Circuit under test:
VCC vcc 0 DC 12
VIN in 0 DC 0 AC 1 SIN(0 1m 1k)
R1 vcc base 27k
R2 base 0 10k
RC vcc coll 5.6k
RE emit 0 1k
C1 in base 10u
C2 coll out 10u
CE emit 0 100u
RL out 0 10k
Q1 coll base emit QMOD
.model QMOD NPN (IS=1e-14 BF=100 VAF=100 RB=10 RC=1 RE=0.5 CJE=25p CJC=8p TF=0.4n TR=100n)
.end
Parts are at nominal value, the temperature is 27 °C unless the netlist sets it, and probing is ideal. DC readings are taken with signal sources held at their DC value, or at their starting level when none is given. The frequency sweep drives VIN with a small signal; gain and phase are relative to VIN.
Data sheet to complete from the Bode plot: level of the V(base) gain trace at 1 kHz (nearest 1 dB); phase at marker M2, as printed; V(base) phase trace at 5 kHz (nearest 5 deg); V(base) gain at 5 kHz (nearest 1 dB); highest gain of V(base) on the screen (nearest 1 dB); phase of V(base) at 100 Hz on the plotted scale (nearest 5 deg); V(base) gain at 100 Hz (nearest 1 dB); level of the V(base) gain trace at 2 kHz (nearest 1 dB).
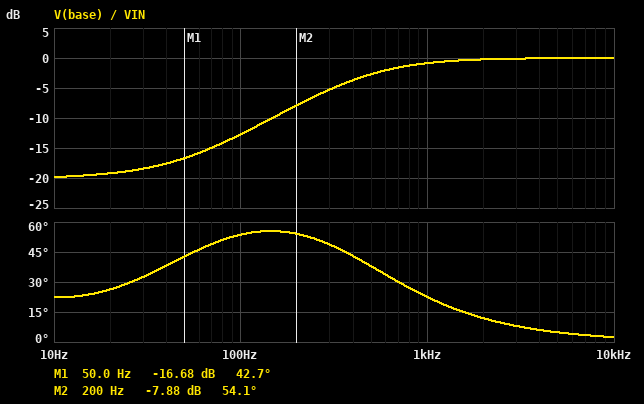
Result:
-1 dB
54.1 deg
5 deg
0 dB
0 dB
55 deg
-13 dB
0 dB
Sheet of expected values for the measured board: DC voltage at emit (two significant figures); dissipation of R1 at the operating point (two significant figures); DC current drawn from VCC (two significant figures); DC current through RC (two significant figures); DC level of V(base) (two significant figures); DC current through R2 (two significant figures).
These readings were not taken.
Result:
1.9 V
3.3 mW
2.1 mA
1.8 mA
2.6 V
260 µA
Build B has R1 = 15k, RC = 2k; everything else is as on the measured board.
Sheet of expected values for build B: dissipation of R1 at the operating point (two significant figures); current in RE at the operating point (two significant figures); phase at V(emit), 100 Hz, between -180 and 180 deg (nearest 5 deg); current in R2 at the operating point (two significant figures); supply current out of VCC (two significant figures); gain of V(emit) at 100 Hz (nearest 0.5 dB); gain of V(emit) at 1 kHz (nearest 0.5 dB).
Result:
3.7 mW
3.9 mA
-20 deg
460 µA
4.3 mA
-1.5 dB
-14.0 dB
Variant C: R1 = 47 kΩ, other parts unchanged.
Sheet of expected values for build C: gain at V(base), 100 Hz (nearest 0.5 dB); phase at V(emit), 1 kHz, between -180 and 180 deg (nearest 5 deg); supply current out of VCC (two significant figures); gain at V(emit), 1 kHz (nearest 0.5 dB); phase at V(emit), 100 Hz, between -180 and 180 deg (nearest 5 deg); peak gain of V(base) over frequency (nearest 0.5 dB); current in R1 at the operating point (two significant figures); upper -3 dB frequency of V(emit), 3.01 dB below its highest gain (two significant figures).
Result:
-0.5 dB
-85 deg
1.5 mA
-22.5 dB
-50 deg
0 dB
210 µA
89 Hz
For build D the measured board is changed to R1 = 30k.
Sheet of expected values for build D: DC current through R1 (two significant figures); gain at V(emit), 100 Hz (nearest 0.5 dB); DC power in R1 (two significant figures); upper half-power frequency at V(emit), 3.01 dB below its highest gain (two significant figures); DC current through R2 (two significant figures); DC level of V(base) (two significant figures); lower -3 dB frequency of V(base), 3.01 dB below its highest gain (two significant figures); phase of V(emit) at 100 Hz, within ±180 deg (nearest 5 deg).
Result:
320 µA
-20.0 dB
3.0 mW
450 Hz
250 µA
2.5 V
440 Hz
-10 deg
